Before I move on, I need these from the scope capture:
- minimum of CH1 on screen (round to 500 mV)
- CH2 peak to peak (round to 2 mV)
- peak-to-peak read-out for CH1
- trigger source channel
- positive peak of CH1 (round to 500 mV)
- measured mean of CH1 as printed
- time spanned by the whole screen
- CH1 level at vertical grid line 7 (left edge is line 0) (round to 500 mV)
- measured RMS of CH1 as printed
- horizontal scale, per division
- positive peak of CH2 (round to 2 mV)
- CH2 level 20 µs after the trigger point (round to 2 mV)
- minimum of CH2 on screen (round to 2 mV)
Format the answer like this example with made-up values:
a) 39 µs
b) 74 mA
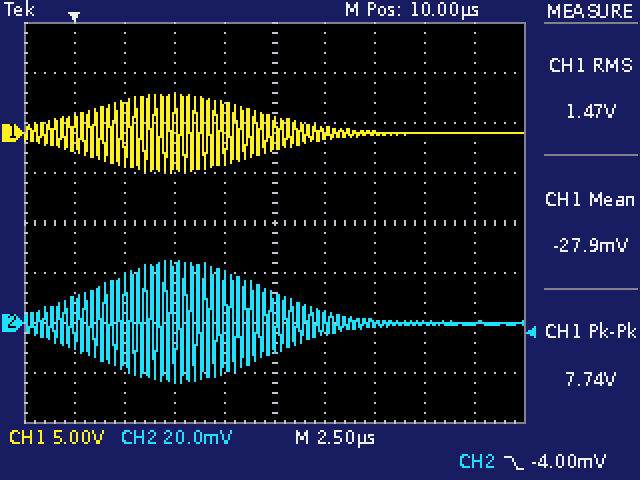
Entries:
a) -4.0 V
b) 48 mV
c) 7.74 V
d) CH2
e) 4.0 V
f) -27.9 mV
g) 25 µs
h) 0.0 V
i) 1.47 V
j) 2.5 µs
k) 24 mV
l) 0 mV
m) -24 mV
